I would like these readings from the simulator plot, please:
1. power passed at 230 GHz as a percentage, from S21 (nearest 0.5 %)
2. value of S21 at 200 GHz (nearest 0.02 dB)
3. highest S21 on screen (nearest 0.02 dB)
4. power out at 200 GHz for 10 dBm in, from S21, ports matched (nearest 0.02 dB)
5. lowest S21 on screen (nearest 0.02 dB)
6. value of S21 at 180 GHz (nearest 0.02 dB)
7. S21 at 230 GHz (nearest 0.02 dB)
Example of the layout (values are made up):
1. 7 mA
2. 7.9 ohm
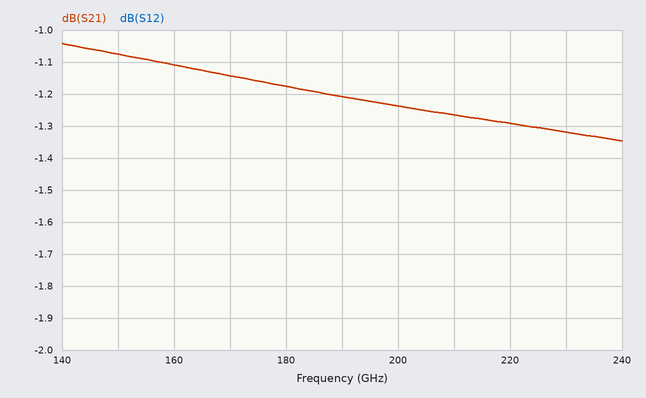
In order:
1. 74.0 %
2. -1.24 dB
3. -1.04 dB
4. 8.76 dBm
5. -1.34 dB
6. -1.18 dB
7. -1.32 dB
